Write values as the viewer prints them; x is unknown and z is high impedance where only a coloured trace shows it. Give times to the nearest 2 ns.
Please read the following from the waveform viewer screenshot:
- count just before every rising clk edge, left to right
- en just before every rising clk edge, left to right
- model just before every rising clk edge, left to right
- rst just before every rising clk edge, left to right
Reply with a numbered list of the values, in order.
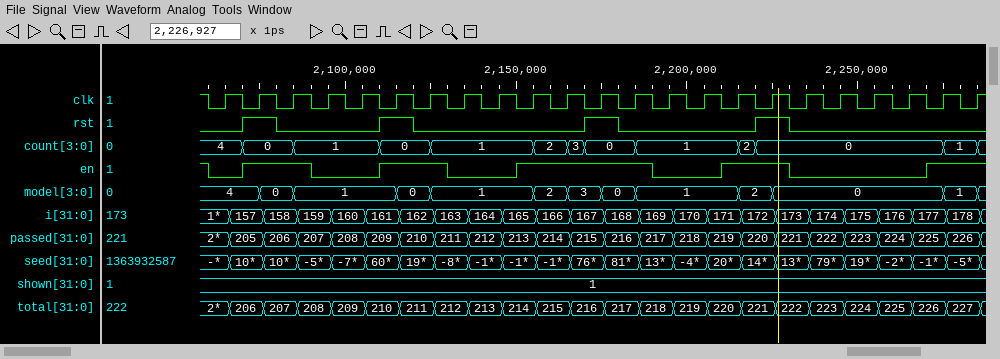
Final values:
1. 4, 0, 0, 1, 1, 0, 0, 1, 1, 1, 2, 0, 0, 1, 1, 1, 0, 0, 0, 0, 0, 0, 1
2. 0 1 1 0 0 1 1 0 0 1 1 1 1 0 0 1 1 0 0 0 0 1 1
3. 4, 4, 0, 1, 1, 1, 0, 1, 1, 1, 2, 3, 0, 1, 1, 1, 2, 0, 0, 0, 0, 0, 1
4. 0 1 0 0 0 1 0 0 0 0 0 1 0 0 0 0 1 0 0 0 0 0 0
